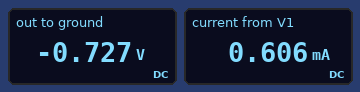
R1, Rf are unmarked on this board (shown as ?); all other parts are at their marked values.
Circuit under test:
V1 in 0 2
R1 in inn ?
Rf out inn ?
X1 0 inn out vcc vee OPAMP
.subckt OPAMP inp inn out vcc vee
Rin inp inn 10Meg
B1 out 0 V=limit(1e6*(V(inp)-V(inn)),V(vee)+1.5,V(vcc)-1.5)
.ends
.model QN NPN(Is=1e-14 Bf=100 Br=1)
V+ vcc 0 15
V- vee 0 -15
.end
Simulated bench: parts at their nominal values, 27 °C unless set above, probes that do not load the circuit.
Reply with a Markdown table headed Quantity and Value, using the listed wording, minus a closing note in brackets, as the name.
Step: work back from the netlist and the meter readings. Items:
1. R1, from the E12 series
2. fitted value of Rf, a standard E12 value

| Quantity | Value |
|---|---|
| R1, from the E12 series | 3.3 kΩ |
| fitted value of Rf, a standard E12 value | 1.2 kΩ |
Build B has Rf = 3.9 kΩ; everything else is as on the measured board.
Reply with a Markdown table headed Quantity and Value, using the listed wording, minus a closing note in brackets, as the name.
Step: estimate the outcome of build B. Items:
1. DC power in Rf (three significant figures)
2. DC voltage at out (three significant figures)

| Quantity | Value |
|---|---|
| DC power in Rf | 1.43 mW |
| DC voltage at out | -2.36 V |
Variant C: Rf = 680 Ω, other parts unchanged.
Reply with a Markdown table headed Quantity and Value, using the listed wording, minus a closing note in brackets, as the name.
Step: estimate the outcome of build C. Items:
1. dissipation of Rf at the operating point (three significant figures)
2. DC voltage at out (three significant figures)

| Quantity | Value |
|---|---|
| dissipation of Rf at the operating point | 250 µW |
| DC voltage at out | -412 mV |
